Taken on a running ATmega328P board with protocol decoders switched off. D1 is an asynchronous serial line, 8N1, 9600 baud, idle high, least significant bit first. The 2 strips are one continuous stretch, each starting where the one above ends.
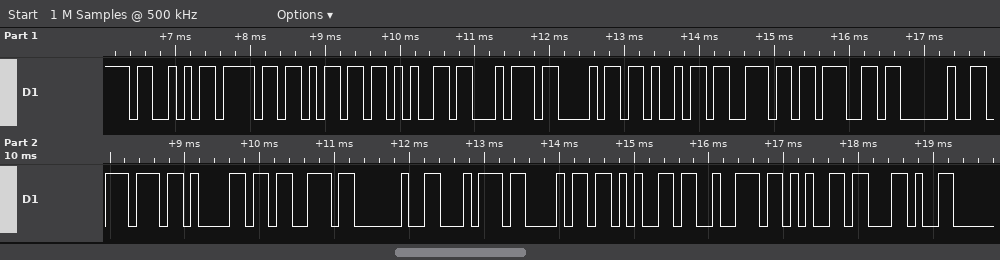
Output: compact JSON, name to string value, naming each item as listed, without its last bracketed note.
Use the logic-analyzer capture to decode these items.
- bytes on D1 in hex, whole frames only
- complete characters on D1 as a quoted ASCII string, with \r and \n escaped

{"bytes on D1 in hex, whole frames only": "0x53 0x6F 0x6D 0x65 0x74 0x68 0x69 0x6E 0x67 0x20 0x77 0x61 0x73 0x20 0x74 0x68 0x65 0x72 0x65 0x2C", "complete characters on D1 as a quoted ASCII string, with \\r and \\n escaped": "\"Something was there,\""}
